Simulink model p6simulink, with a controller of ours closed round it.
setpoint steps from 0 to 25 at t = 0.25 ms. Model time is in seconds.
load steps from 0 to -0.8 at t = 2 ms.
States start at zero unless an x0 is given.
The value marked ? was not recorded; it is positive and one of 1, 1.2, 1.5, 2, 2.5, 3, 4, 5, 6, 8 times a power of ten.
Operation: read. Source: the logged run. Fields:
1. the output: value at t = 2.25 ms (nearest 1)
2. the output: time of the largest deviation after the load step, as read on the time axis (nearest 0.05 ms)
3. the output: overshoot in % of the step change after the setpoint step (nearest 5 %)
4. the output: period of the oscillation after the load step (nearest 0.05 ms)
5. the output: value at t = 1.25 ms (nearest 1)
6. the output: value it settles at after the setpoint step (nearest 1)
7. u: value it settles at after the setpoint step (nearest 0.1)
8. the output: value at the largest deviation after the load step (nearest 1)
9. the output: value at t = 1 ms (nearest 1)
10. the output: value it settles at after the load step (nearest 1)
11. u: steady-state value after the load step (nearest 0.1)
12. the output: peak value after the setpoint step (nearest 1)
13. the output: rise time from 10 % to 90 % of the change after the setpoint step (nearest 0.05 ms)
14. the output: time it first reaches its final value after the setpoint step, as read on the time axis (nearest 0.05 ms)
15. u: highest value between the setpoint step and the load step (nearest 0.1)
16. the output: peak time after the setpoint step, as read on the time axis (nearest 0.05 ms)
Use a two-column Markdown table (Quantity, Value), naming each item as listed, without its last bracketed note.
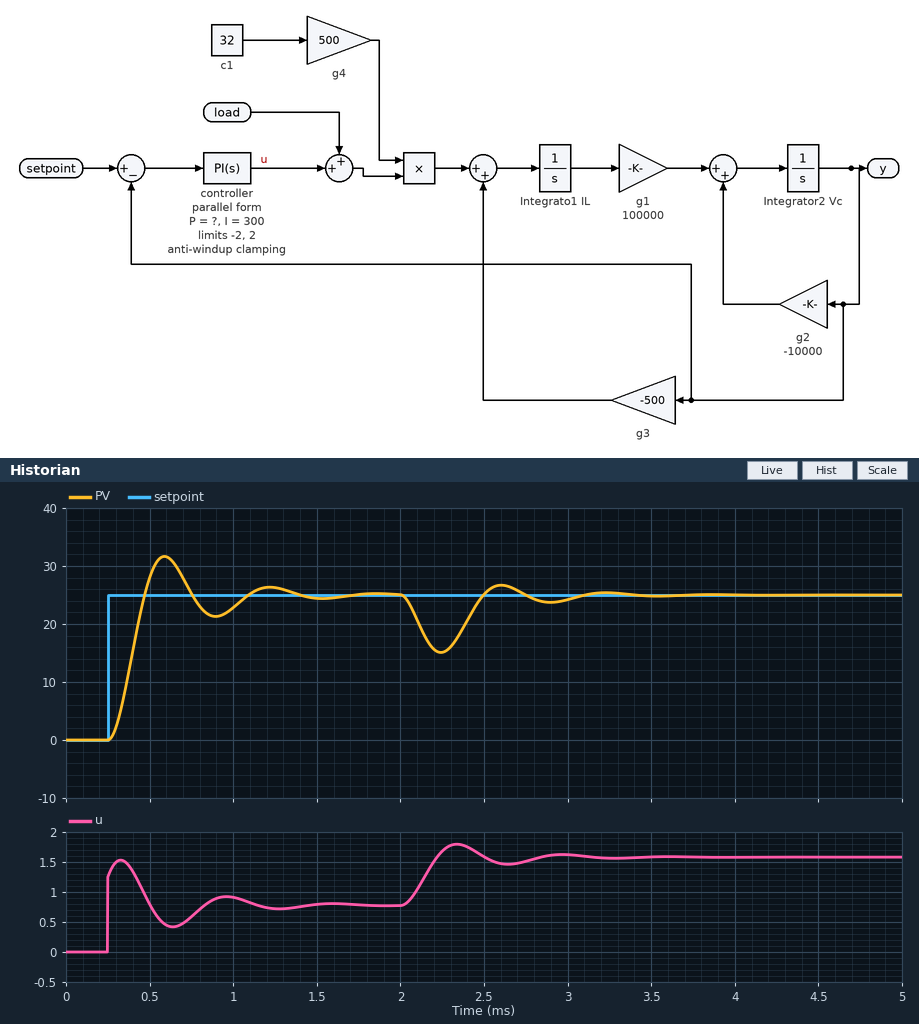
| Quantity | Value |
|---|---|
| the output: value at t = 2.25 ms | 15 |
| the output: time of the largest deviation after the load step, as read on the time axis | 2.25 ms |
| the output: overshoot in % of the step change after the setpoint step | 25 % |
| the output: period of the oscillation after the load step | 0.65 ms |
| the output: value at t = 1.25 ms | 26 |
| the output: value it settles at after the setpoint step | 25 |
| u: value it settles at after the setpoint step | 0.8 |
| the output: value at the largest deviation after the load step | 15 |
| the output: value at t = 1 ms | 23 |
| the output: value it settles at after the load step | 25 |
| u: steady-state value after the load step | 1.6 |
| the output: peak value after the setpoint step | 32 |
| the output: rise time from 10 % to 90 % of the change after the setpoint step | 0.15 ms |
| the output: time it first reaches its final value after the setpoint step, as read on the time axis | 0.45 ms |
| u: highest value between the setpoint step and the load step | 1.5 |
| the output: peak time after the setpoint step, as read on the time axis | 0.60 ms |
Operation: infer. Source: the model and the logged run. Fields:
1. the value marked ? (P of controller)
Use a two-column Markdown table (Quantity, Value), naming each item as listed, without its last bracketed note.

| Quantity | Value |
|---|---|
| the value marked ? | 0.05 |
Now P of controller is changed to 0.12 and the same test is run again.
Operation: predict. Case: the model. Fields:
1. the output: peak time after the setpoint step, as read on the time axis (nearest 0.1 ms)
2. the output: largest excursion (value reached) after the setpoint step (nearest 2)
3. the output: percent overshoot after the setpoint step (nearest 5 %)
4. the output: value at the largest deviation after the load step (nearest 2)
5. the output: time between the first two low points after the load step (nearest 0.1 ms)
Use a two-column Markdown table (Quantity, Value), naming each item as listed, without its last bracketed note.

| Quantity | Value |
|---|---|
| the output: peak time after the setpoint step, as read on the time axis | 0.5 ms |
| the output: largest excursion (value reached) after the setpoint step | 28 |
| the output: percent overshoot after the setpoint step | 10 % |
| the output: value at the largest deviation after the load step | 18 |
| the output: time between the first two low points after the load step | 0.4 ms |
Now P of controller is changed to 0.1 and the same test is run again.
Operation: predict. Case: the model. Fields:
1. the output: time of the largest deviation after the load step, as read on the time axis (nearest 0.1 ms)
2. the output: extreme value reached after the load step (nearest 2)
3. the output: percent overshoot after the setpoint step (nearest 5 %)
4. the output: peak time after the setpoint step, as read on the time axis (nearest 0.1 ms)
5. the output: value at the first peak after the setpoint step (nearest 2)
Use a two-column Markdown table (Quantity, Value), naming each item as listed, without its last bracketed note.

| Quantity | Value |
|---|---|
| the output: time of the largest deviation after the load step, as read on the time axis | 2.2 ms |
| the output: extreme value reached after the load step | 18 |
| the output: percent overshoot after the setpoint step | 10 % |
| the output: peak time after the setpoint step, as read on the time axis | 0.5 ms |
| the output: value at the first peak after the setpoint step | 28 |
